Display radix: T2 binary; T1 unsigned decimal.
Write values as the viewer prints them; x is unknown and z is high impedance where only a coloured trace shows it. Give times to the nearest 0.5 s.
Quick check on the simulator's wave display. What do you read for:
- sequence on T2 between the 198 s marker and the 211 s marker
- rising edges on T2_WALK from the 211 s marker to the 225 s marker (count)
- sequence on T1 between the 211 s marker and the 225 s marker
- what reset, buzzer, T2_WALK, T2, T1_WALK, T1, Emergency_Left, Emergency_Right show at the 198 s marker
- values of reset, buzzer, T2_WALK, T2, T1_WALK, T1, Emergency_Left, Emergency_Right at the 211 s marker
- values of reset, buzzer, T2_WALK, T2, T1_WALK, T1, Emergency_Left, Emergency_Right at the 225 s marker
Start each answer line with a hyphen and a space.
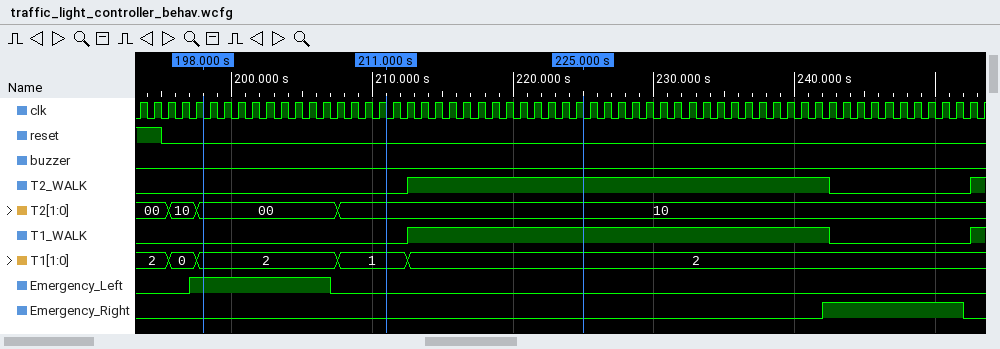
- 00, 10
- 1
- 1, 2
- reset=0, buzzer=0, T2_WALK=0, T2=00, T1_WALK=0, T1=2, Emergency_Left=1, Emergency_Right=0
- reset=0, buzzer=0, T2_WALK=0, T2=10, T1_WALK=0, T1=1, Emergency_Left=0, Emergency_Right=0
- reset=0, buzzer=0, T2_WALK=1, T2=10, T1_WALK=1, T1=2, Emergency_Left=0, Emergency_Right=0
